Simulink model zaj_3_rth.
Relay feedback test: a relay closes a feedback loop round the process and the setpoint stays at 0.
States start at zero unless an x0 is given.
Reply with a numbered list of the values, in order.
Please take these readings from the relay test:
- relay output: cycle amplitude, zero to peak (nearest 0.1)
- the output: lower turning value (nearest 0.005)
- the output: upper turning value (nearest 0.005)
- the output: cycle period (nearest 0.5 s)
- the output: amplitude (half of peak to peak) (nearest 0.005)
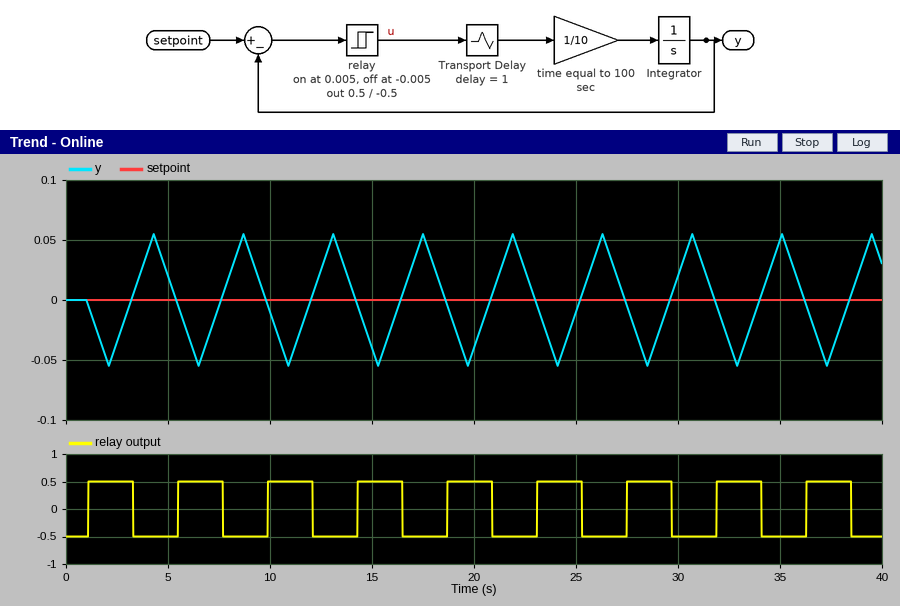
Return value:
1. 0.5
2. -0.055
3. 0.055
4. 4.5 s
5. 0.055
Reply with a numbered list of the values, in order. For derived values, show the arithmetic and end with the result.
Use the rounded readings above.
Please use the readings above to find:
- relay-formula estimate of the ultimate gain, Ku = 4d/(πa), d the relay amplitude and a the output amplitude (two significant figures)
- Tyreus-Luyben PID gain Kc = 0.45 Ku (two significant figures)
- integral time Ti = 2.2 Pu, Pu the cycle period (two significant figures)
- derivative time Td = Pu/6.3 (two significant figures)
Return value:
1. 4 × 0.5 / (π × 0.055) = 12
2. 0.45 × 12 = 5.4
3. 2.2 × 4.5 = 9.9 s
4. 4.5 / 6.3 = 0.71 s
